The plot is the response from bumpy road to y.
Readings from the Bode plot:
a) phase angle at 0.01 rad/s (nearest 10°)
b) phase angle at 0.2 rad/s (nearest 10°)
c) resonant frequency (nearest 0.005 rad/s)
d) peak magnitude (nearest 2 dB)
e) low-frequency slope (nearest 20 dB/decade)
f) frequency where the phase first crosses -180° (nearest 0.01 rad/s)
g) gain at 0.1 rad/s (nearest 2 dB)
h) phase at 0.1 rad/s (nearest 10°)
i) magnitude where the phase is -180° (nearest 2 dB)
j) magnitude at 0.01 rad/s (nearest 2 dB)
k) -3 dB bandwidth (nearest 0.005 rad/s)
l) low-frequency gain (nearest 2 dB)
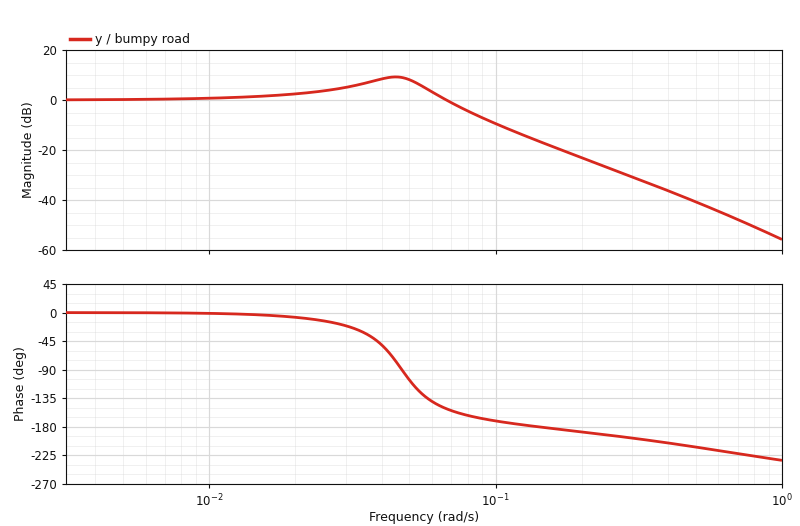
0°
-190°
0.045 rad/s
10 dB
0 dB/decade
0.14 rad/s
-10 dB
-170°
-16 dB
0 dB
0.075 rad/s
0 dB
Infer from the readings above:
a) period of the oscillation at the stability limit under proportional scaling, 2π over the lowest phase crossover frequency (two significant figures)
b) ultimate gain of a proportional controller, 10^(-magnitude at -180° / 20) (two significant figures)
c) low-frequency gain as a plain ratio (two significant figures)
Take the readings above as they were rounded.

45 s
6.3
1.0
